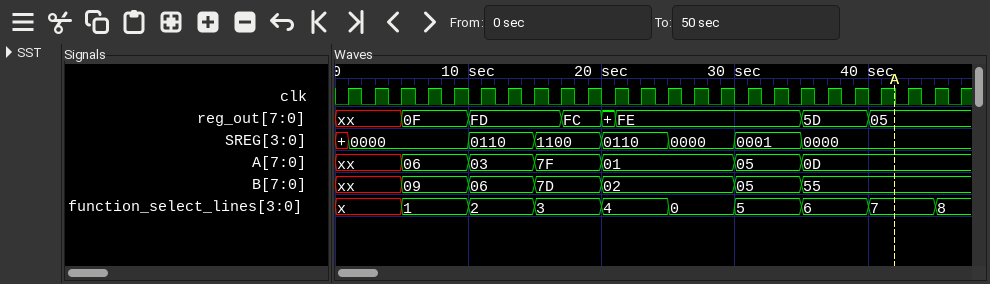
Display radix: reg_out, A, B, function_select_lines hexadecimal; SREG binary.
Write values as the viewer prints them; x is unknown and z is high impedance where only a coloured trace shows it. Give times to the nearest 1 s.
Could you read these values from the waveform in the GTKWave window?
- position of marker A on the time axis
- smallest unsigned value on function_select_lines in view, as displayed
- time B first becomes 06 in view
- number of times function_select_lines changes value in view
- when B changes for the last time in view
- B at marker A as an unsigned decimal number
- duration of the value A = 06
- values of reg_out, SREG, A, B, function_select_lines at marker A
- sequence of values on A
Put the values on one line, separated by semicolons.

42 s; 0; 10 s; 9; 35 s; 85; 5 s; reg_out=05, SREG=0000, A=0D, B=55, function_select_lines=7; xx, 06, 03, 7F, 01, 05, 0D
